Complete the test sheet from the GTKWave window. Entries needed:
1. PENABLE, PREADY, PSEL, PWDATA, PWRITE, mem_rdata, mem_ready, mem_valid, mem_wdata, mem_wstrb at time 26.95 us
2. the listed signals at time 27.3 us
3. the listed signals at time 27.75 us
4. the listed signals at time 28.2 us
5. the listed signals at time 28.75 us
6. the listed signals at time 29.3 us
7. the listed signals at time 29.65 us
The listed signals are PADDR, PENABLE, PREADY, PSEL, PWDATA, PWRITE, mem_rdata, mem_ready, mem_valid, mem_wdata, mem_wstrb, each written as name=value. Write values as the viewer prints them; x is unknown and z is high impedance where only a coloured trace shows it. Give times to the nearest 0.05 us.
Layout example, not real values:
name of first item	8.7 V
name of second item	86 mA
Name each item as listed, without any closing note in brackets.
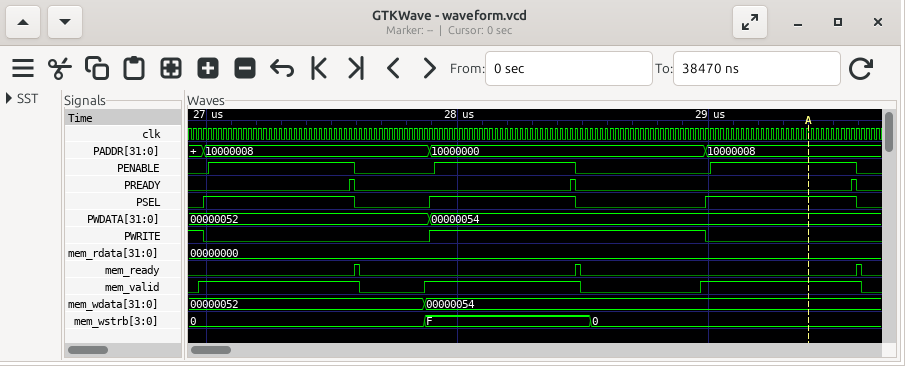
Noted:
PENABLE, PREADY, PSEL, PWDATA, PWRITE, mem_rdata, mem_ready, mem_valid, mem_wdata, mem_wstrb at time 26.95 us	PENABLE=0, PREADY=0, PSEL=0, PWDATA=00000052, PWRITE=1, mem_rdata=00000000, mem_ready=0, mem_valid=0, mem_wdata=00000052, mem_wstrb=0
the listed signals at time 27.3 us	PADDR=10000008, PENABLE=1, PREADY=0, PSEL=1, PWDATA=00000052, PWRITE=0, mem_rdata=00000000, mem_ready=0, mem_valid=1, mem_wdata=00000052, mem_wstrb=0
the listed signals at time 27.75 us	PADDR=10000008, PENABLE=0, PREADY=0, PSEL=0, PWDATA=00000052, PWRITE=0, mem_rdata=00000000, mem_ready=0, mem_valid=0, mem_wdata=00000052, mem_wstrb=0
the listed signals at time 28.2 us	PADDR=10000000, PENABLE=1, PREADY=0, PSEL=1, PWDATA=00000054, PWRITE=1, mem_rdata=00000000, mem_ready=0, mem_valid=1, mem_wdata=00000054, mem_wstrb=F
the listed signals at time 28.75 us	PADDR=10000000, PENABLE=0, PREADY=0, PSEL=0, PWDATA=00000054, PWRITE=1, mem_rdata=00000000, mem_ready=0, mem_valid=0, mem_wdata=00000054, mem_wstrb=0
the listed signals at time 29.3 us	PADDR=10000008, PENABLE=1, PREADY=0, PSEL=1, PWDATA=00000054, PWRITE=0, mem_rdata=00000000, mem_ready=0, mem_valid=1, mem_wdata=00000054, mem_wstrb=0
the listed signals at time 29.65 us	PADDR=10000008, PENABLE=0, PREADY=0, PSEL=0, PWDATA=00000054, PWRITE=0, mem_rdata=00000000, mem_ready=0, mem_valid=0, mem_wdata=00000054, mem_wstrb=0
